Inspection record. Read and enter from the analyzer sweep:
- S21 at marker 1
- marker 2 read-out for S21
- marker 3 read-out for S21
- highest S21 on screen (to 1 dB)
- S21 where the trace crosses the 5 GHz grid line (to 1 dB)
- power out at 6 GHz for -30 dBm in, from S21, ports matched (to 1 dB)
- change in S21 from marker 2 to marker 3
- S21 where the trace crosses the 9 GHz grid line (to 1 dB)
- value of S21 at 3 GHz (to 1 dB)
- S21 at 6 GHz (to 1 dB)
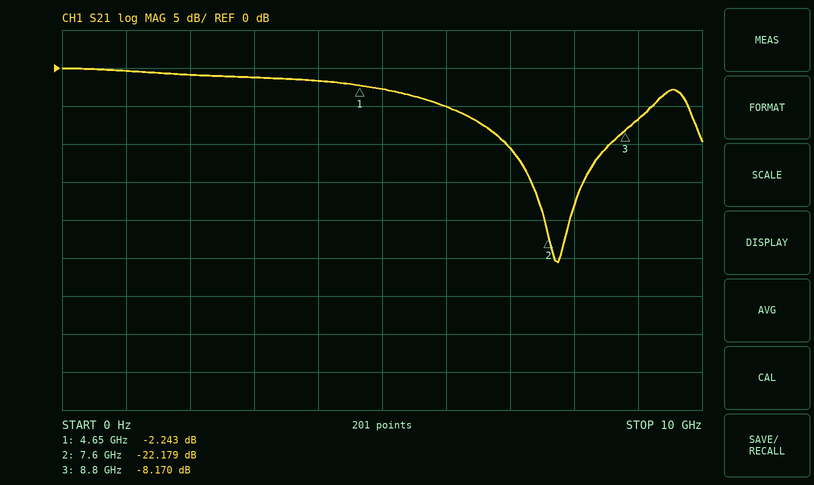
-2.243 dB
-22.179 dB
-8.170 dB
0 dB
-3 dB
-35 dBm
14.009 dB
-7 dB
-1 dB
-5 dB
